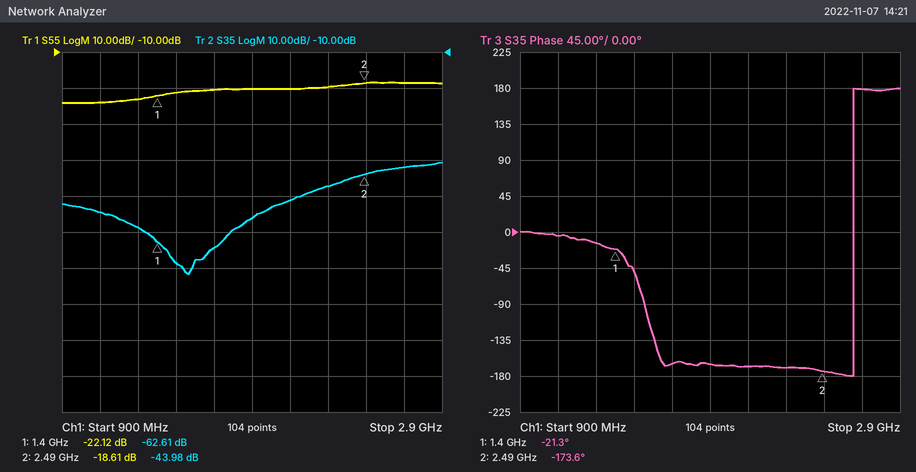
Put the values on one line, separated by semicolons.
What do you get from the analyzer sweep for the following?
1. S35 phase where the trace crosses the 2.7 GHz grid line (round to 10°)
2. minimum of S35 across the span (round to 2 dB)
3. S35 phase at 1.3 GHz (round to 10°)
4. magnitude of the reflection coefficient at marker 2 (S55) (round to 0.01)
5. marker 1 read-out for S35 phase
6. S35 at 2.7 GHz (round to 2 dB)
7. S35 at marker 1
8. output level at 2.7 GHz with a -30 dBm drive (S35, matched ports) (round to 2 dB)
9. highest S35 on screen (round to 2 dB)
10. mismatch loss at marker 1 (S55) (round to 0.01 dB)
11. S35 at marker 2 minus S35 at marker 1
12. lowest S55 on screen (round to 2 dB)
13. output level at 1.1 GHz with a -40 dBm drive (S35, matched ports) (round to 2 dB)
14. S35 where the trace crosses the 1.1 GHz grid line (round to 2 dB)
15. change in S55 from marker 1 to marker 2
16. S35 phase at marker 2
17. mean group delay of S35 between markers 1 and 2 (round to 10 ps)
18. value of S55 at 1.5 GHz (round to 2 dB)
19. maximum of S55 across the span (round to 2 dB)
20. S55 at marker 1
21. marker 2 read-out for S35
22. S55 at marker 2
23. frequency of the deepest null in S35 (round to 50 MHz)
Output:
180°; -72 dB; -10°; 0.12; -21.3°; -42 dB; -62.61 dB; -72 dBm; -40 dB; 0.03 dB; 18.63 dB; -24 dB; -94 dBm; -54 dB; 3.51 dB; -173.6°; 390 ps; -22 dB; -18 dB; -22.12 dB; -43.98 dB; -18.61 dB; 1.55 GHz
